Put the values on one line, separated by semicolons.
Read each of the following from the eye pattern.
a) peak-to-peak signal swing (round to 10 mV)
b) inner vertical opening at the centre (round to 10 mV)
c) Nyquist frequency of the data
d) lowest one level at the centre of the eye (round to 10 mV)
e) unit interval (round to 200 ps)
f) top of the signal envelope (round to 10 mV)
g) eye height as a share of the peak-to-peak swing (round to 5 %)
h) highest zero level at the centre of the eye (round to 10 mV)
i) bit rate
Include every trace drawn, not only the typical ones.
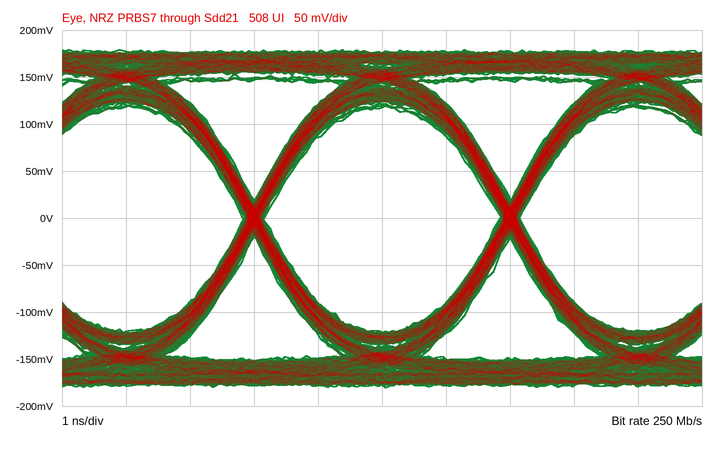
360 mV; 240 mV; 125 MHz; 120 mV; 4.0 ns; 180 mV; 65 %; -120 mV; 250 Mb/s
